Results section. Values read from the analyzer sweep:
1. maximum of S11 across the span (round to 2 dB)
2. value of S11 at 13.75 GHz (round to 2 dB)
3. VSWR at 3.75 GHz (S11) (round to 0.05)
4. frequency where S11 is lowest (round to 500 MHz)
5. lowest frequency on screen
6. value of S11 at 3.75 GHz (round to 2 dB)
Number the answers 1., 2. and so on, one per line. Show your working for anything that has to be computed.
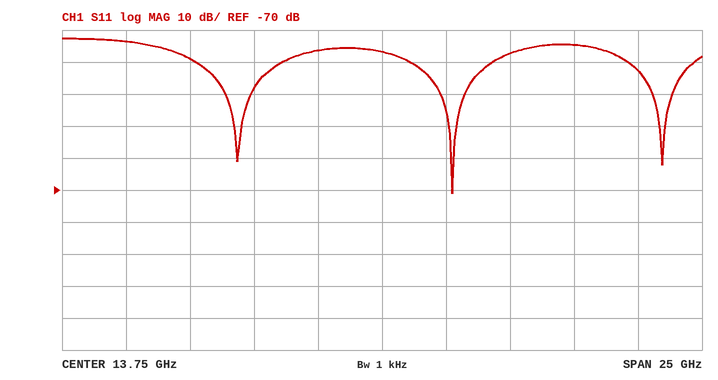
1. -22 dB
2. -26 dB
3. |Γ| = 10^(-24/20) = 0.0631; VSWR = (1 + 0.0631)/(1 − 0.0631) ≈ 1.13, so 1.15 to the nearest 0.05
4. 16.5 GHz
5. 1.25 GHz
6. -24 dB
